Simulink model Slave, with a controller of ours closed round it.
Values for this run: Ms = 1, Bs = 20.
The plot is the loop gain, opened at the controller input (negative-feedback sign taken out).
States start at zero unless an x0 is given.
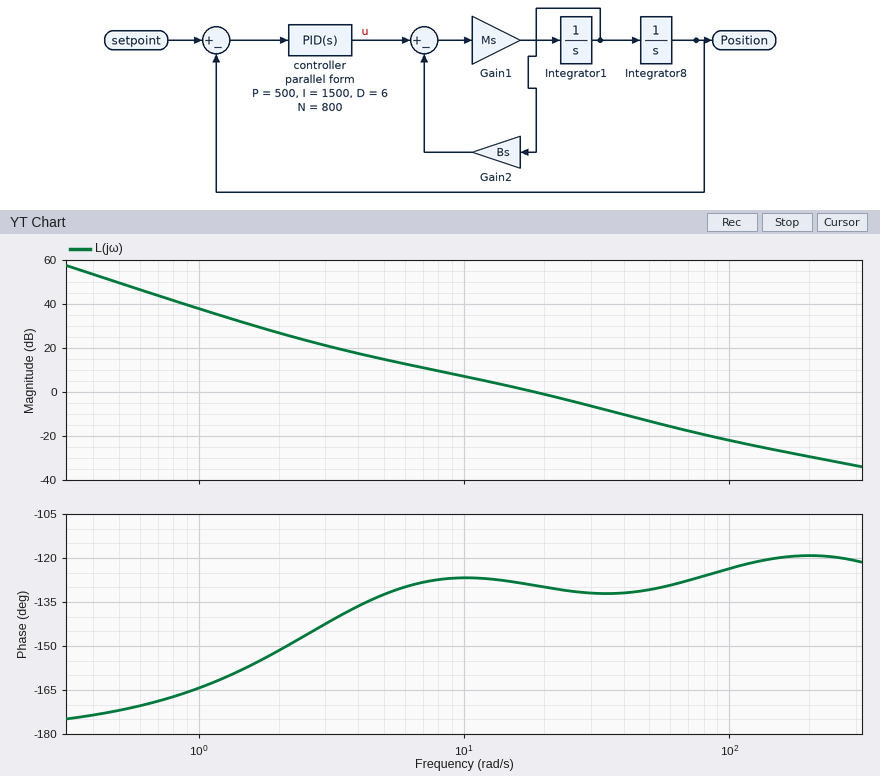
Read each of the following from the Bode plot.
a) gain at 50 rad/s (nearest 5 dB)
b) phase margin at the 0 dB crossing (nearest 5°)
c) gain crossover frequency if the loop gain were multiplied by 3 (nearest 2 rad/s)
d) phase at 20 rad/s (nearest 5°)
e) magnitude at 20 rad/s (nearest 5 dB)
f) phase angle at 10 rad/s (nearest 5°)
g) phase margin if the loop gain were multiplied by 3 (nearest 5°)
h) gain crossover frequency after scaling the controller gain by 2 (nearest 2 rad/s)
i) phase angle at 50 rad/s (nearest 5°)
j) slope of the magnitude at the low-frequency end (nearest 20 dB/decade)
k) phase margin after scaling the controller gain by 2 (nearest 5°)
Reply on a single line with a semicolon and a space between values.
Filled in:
-15 dB; 50°; 38 rad/s; -130°; 0 dB; -125°; 50°; 30 rad/s; -130°; -40 dB/decade; 50°
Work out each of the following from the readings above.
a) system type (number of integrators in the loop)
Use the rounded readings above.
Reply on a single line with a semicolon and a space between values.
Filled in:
2
